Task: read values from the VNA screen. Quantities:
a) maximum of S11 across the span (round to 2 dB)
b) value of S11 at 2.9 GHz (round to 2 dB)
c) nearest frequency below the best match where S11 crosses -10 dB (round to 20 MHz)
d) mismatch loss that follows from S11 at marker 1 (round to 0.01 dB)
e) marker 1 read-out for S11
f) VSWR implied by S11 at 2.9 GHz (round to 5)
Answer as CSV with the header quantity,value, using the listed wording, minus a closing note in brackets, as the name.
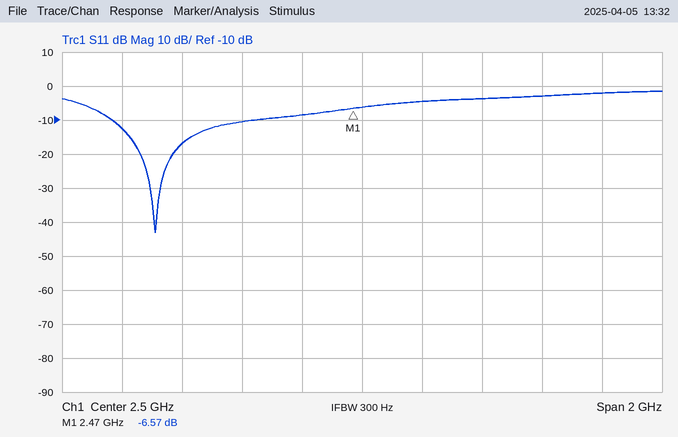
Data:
quantity,value
maximum of S11 across the span,-2 dB
value of S11 at 2.9 GHz,-4 dB
nearest frequency below the best match where S11 crosses -10 dB,1.66 GHz
mismatch loss that follows from S11 at marker 1,1.08 dB
marker 1 read-out for S11,-6.57 dB
VSWR implied by S11 at 2.9 GHz,5
